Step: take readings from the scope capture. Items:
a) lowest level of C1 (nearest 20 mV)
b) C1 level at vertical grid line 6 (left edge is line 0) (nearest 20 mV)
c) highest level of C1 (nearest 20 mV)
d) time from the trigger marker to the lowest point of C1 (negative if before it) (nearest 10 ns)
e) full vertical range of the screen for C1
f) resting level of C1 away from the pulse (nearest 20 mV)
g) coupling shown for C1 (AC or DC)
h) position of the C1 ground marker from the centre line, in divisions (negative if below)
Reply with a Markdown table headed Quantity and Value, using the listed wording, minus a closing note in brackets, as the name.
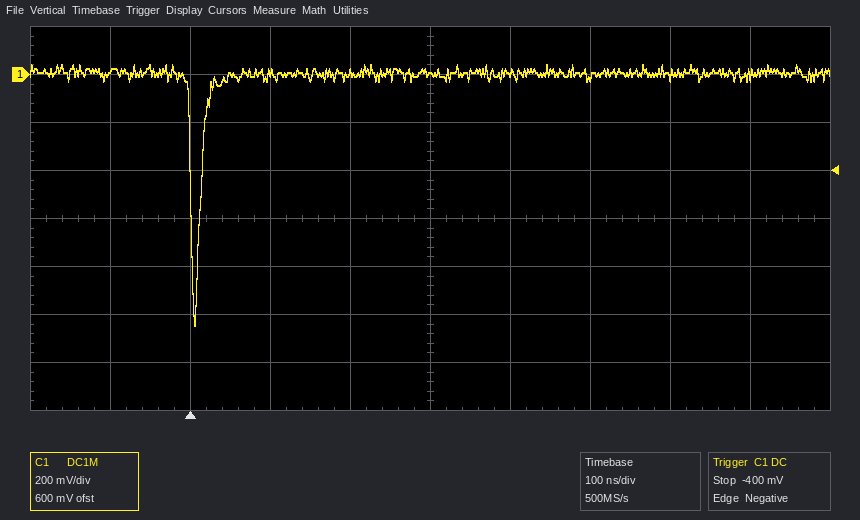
| Quantity | Value |
|---|---|
| lowest level of C1 | -1.04 V |
| C1 level at vertical grid line 6 (left edge is line 0) | 0 mV |
| highest level of C1 | 40 mV |
| time from the trigger marker to the lowest point of C1 (negative if before it) | +10 ns |
| full vertical range of the screen for C1 | 1.6 V |
| resting level of C1 away from the pulse | 0 mV |
| coupling shown for C1 | DC |
| position of the C1 ground marker from the centre line, in divisions | +3.0 div |
